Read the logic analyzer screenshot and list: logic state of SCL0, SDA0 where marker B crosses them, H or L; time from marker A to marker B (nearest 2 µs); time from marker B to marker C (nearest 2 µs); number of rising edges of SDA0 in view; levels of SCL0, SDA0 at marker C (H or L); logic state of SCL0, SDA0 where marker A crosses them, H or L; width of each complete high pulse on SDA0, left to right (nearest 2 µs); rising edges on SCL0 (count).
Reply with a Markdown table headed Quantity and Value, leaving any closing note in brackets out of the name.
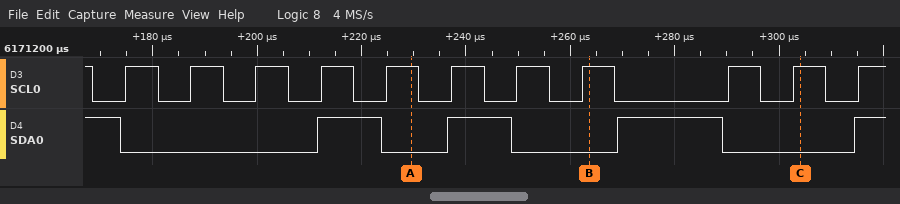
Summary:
| Quantity | Value |
|---|---|
| logic state of SCL0, SDA0 where marker B crosses them, H or L | SCL0=H, SDA0=L |
| time from marker A to marker B | 34 µs |
| time from marker B to marker C | 40 µs |
| number of rising edges of SDA0 in view | 4 |
| levels of SCL0, SDA0 at marker C | SCL0=H, SDA0=L |
| logic state of SCL0, SDA0 where marker A crosses them, H or L | SCL0=H, SDA0=L |
| width of each complete high pulse on SDA0, left to right | 12 µs, 12 µs, 20 µs |
| rising edges on SCL0 | 11 |
